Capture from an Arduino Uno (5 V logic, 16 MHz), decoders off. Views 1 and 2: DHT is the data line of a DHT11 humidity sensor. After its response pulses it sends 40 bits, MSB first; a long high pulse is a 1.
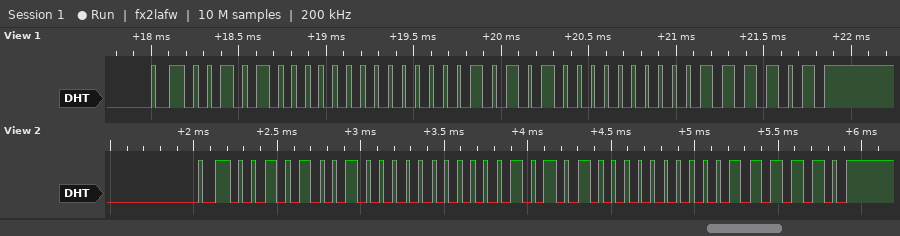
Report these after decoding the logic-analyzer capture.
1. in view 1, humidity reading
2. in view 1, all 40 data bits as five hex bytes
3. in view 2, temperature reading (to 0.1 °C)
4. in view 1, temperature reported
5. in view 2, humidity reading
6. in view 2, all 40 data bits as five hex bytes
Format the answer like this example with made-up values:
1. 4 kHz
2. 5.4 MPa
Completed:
1. 40 %
2. 28 00 15 00 3D
3. 21.0 °C
4. 21.0 °C
5. 41 %
6. 29 00 15 00 3E
